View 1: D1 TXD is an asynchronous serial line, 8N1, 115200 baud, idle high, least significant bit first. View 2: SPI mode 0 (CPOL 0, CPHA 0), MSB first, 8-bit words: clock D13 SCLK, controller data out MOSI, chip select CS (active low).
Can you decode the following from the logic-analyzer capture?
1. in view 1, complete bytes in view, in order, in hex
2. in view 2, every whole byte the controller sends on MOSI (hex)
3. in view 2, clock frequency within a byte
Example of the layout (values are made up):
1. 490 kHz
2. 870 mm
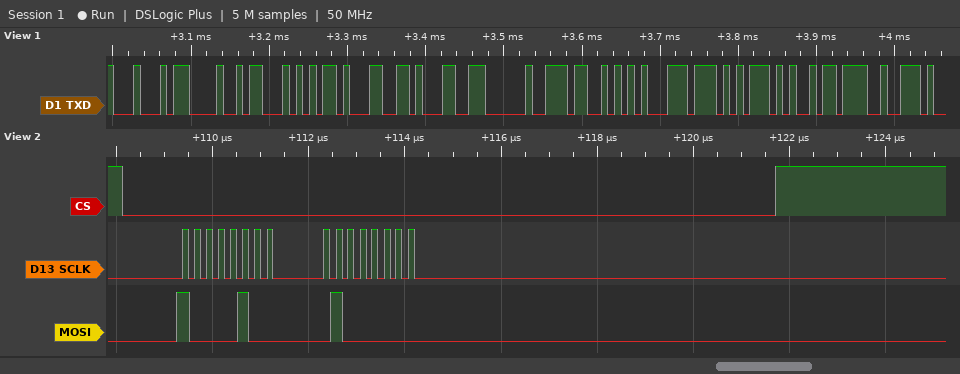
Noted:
1. 44 48 54 31 31 20 53 71 75 69 72
2. 84 40
3. 4 MHz
